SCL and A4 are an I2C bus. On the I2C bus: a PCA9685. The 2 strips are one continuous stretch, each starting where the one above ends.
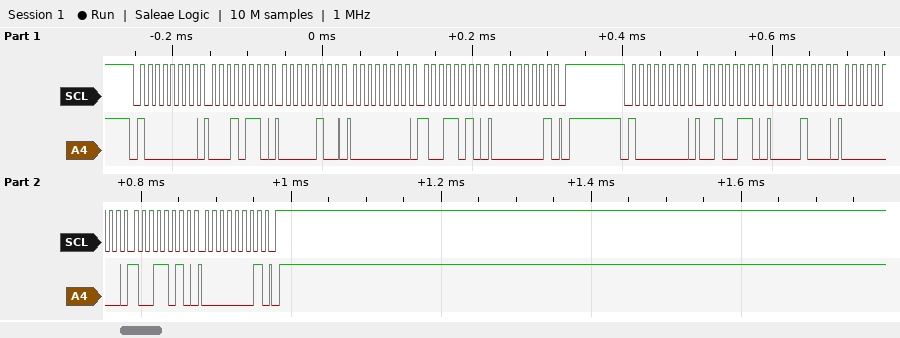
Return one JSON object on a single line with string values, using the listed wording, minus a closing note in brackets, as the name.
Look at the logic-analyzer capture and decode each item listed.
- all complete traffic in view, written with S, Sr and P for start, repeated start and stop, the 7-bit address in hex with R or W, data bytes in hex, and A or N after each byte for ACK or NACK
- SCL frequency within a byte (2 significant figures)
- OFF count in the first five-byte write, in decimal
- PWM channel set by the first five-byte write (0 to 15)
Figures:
{"all complete traffic in view, written with S, Sr and P for start, repeated start and stop, the 7-bit address in hex with R or W, data bytes in hex, and A or N after each byte for ACK or NACK": "S 40W A 16 A 04 A 00 A 9A A 01 A P S 40W A 26 A 08 A 00 A 9A A 01 A P", "SCL frequency within a byte": "100 kHz", "OFF count in the first five-byte write, in decimal": "410", "PWM channel set by the first five-byte write": "4"}
